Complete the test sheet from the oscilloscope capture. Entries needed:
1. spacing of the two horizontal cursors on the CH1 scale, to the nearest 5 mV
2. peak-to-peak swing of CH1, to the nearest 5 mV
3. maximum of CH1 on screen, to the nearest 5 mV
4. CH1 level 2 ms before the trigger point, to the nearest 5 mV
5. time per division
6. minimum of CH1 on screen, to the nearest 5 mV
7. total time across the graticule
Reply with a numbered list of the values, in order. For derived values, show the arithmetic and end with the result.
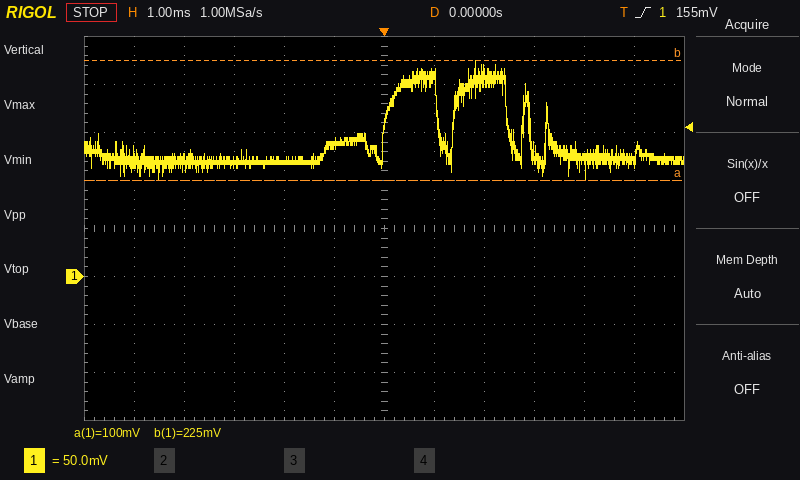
1. 125 mV
2. 225 mV − (100 mV) = 125 mV
3. 225 mV
4. 120 mV
5. 1 ms
6. 100 mV
7. 12 ms
